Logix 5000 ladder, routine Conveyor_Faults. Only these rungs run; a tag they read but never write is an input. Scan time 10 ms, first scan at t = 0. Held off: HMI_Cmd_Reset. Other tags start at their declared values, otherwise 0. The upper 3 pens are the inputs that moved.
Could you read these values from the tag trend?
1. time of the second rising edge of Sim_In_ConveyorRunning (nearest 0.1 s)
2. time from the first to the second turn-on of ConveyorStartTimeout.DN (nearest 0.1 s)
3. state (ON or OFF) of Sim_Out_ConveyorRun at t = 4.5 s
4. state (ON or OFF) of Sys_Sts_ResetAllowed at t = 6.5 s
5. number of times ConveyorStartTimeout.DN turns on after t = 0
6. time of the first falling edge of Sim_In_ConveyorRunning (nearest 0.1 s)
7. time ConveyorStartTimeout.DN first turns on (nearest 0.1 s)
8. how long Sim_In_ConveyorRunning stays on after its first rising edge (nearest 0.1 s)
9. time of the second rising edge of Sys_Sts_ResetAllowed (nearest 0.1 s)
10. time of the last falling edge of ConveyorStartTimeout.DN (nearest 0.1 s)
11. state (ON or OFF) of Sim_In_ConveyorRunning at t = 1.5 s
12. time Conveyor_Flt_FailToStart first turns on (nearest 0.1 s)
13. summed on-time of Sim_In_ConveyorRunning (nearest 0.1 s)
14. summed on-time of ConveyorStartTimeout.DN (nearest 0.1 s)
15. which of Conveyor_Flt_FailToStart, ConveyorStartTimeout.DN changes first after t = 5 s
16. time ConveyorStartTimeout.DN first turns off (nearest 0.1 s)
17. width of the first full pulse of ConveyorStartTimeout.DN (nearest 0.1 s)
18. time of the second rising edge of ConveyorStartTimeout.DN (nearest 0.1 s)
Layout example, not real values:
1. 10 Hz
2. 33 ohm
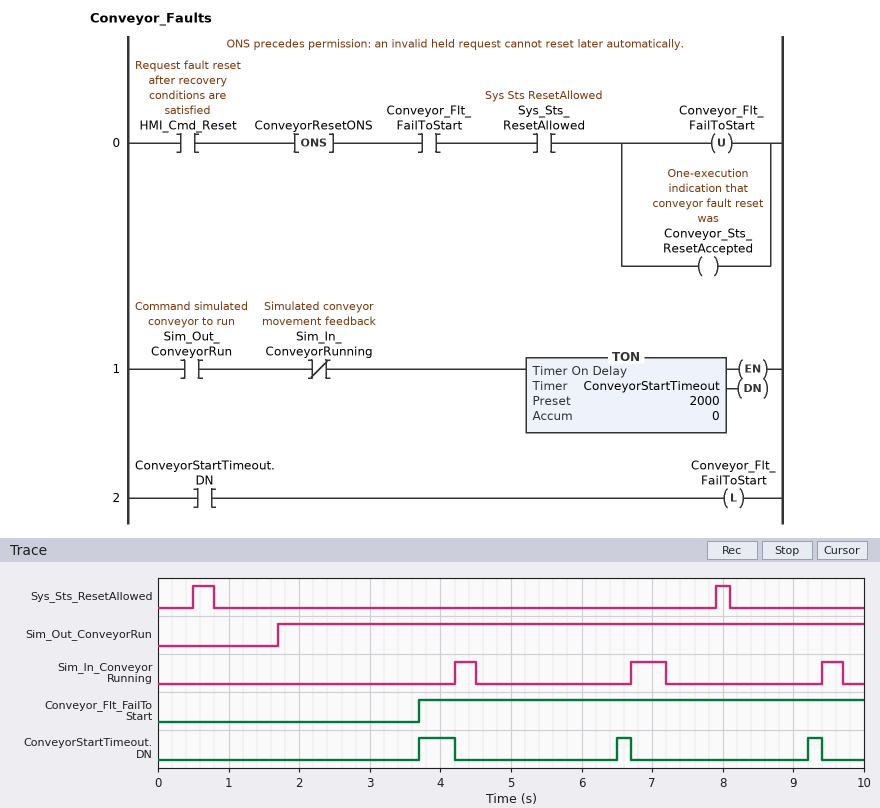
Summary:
1. 6.7 s
2. 2.8 s
3. ON
4. OFF
5. 3
6. 4.5 s
7. 3.7 s
8. 0.3 s
9. 7.9 s
10. 9.4 s
11. OFF
12. 3.7 s
13. 1.1 s
14. 0.9 s
15. ConveyorStartTimeout.DN
16. 4.2 s
17. 0.5 s
18. 6.5 s
